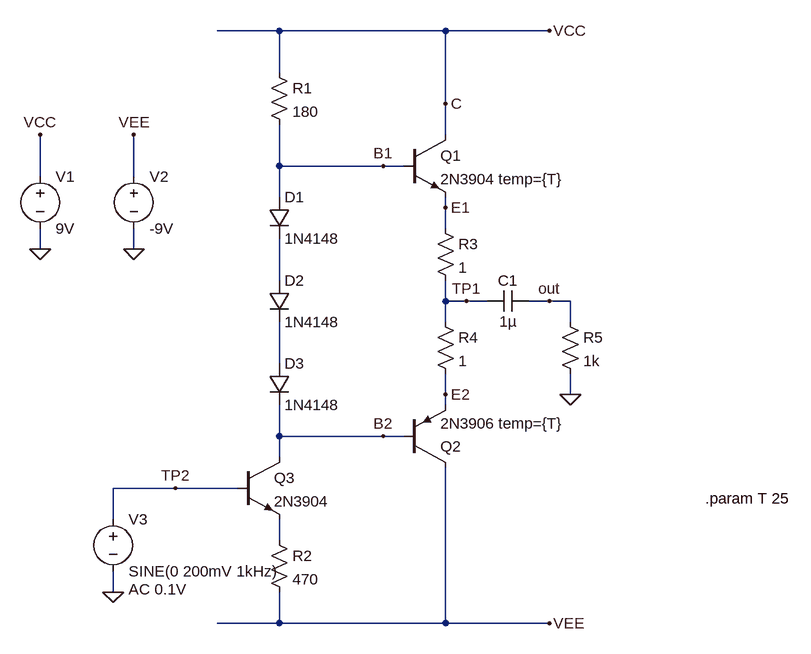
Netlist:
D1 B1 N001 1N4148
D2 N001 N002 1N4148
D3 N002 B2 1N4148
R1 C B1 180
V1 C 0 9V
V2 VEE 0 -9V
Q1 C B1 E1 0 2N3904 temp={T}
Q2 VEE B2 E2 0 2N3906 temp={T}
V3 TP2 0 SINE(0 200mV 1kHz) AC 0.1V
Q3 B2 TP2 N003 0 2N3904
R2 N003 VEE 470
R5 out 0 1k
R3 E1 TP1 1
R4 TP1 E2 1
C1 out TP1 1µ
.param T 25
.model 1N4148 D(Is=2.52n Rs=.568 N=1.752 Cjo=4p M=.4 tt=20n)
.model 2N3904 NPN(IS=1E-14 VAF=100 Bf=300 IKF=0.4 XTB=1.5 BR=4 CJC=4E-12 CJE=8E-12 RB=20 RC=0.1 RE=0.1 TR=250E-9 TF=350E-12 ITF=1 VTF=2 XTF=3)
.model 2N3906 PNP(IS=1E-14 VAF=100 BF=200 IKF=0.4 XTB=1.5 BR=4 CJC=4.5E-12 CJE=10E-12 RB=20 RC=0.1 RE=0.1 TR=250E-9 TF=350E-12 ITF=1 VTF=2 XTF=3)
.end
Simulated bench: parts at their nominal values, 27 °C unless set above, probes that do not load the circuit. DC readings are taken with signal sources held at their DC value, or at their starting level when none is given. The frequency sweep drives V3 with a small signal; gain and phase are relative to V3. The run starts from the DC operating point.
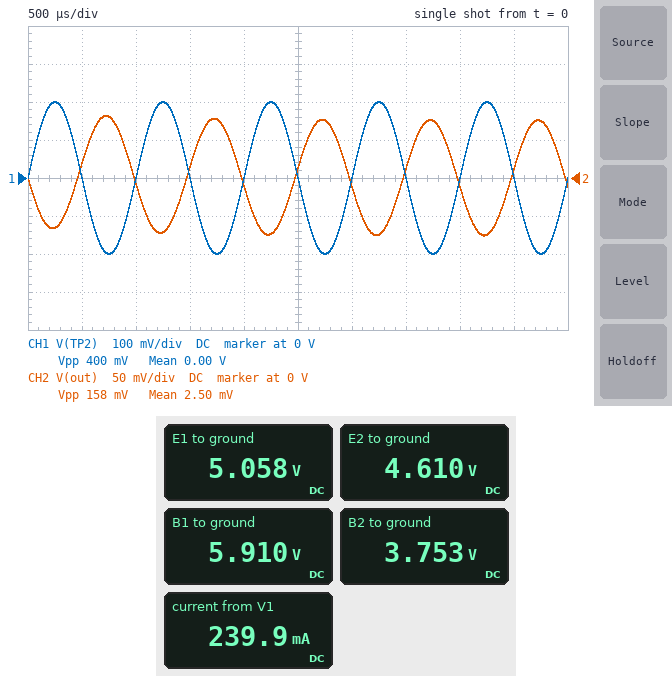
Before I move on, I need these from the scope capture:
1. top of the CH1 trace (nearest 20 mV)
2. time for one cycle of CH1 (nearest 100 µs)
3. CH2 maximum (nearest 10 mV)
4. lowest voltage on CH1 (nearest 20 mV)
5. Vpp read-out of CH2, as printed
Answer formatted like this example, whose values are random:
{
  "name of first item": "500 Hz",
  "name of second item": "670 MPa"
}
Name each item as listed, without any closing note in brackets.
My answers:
{
  "top of the CH1 trace": "200 mV",
  "time for one cycle of CH1": "1.0 ms",
  "CH2 maximum": "80 mV",
  "lowest voltage on CH1": "-200 mV",
  "Vpp read-out of CH2, as printed": "158 mV"
}
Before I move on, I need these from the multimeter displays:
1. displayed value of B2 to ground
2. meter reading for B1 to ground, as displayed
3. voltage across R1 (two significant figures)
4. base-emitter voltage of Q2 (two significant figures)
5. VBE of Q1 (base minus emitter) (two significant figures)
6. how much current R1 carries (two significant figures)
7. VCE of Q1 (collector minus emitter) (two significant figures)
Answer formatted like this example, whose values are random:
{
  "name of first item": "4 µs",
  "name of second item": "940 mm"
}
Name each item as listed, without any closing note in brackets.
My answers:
{
  "displayed value of B2 to ground": "3.753 V",
  "meter reading for B1 to ground, as displayed": "5.910 V",
  "voltage across R1": "3.1 V",
  "base-emitter voltage of Q2": "-860 mV",
  "VBE of Q1 (base minus emitter)": "850 mV",
  "how much current R1 carries": "17 mA",
  "VCE of Q1 (collector minus emitter)": "3.9 V"
}
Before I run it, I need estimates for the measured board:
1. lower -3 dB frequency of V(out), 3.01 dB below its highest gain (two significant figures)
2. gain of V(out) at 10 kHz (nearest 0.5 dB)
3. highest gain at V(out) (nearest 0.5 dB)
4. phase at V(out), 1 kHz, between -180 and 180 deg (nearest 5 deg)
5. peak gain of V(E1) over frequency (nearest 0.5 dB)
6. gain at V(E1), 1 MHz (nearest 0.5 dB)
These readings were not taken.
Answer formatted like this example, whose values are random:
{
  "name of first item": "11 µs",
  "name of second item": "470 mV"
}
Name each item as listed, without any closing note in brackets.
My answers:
{
  "lower -3 dB frequency of V(out), 3.01 dB below its highest gain": "160 Hz",
  "gain of V(out) at 10 kHz": "-8.5 dB",
  "highest gain at V(out)": "-8.5 dB",
  "phase at V(out), 1 kHz, between -180 and 180 deg": "-170 deg",
  "peak gain of V(E1) over frequency": "-8.5 dB",
  "gain at V(E1), 1 MHz": "-8.5 dB"
}
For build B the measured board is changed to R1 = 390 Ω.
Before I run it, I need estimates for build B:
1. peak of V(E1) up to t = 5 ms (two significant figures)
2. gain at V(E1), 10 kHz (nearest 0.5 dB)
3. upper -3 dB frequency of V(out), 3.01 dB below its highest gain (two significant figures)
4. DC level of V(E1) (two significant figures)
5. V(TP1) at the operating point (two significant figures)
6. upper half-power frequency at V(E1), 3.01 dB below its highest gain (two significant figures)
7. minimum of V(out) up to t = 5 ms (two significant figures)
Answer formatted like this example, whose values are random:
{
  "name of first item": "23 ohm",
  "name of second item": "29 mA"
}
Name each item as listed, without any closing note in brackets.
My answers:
{
  "peak of V(E1) up to t = 5 ms": "1.7 V",
  "gain at V(E1), 10 kHz": "-2.0 dB",
  "upper -3 dB frequency of V(out), 3.01 dB below its highest gain": "85 MHz",
  "DC level of V(E1)": "1.5 V",
  "V(TP1) at the operating point": "1.3 V",
  "upper half-power frequency at V(E1), 3.01 dB below its highest gain": "87 MHz",
  "minimum of V(out) up to t = 5 ms": "-160 mV"
}
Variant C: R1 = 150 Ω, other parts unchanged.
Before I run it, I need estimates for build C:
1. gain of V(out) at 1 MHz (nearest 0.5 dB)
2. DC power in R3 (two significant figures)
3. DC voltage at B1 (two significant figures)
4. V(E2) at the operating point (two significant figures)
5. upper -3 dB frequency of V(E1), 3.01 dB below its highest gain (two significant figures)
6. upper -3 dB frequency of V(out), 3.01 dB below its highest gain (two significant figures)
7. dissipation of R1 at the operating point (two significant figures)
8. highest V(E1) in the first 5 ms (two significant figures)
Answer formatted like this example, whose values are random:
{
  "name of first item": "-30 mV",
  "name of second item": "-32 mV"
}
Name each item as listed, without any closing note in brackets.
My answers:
{
  "gain of V(out) at 1 MHz": "-10.0 dB",
  "DC power in R3": "50 mW",
  "DC voltage at B1": "6.4 V",
  "V(E2) at the operating point": "5.1 V",
  "upper -3 dB frequency of V(E1), 3.01 dB below its highest gain": "3.5 GHz",
  "upper -3 dB frequency of V(out), 3.01 dB below its highest gain": "3.4 GHz",
  "dissipation of R1 at the operating point": "44 mW",
  "highest V(E1) in the first 5 ms": "5.6 V"
}
